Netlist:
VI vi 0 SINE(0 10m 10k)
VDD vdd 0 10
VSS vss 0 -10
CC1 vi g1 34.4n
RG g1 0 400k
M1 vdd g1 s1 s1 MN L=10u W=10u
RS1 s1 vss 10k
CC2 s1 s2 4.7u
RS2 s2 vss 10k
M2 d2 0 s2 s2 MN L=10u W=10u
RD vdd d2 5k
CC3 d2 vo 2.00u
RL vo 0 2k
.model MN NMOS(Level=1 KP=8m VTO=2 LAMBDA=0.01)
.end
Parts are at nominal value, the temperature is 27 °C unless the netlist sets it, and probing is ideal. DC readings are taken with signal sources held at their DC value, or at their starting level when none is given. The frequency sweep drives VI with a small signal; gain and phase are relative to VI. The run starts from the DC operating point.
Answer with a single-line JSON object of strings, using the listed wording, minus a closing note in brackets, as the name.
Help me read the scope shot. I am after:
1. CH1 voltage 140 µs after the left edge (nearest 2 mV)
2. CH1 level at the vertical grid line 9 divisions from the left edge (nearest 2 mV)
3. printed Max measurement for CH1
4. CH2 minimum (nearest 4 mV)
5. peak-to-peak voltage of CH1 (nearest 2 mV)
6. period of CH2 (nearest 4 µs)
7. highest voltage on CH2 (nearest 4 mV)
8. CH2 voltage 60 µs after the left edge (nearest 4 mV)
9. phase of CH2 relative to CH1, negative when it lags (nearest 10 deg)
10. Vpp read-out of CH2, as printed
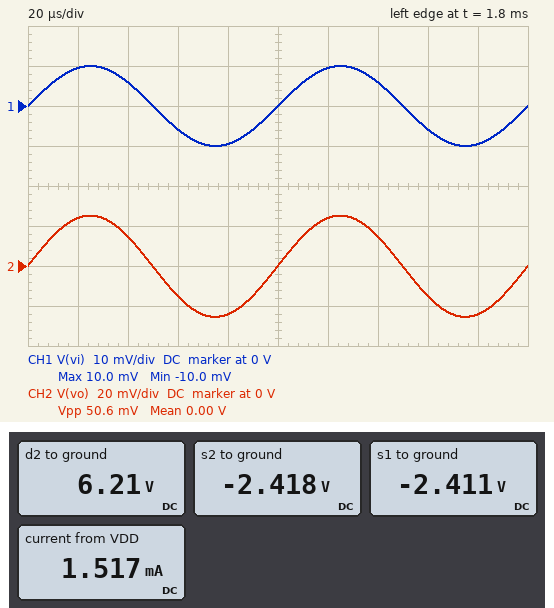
{"CH1 voltage 140 µs after the left edge": "6 mV", "CH1 level at the vertical grid line 9 divisions from the left edge": "-10 mV", "printed Max measurement for CH1": "10.0 mV", "CH2 minimum": "-24 mV", "peak-to-peak voltage of CH1": "20 mV", "period of CH2": "100 µs", "highest voltage on CH2": "24 mV", "CH2 voltage 60 µs after the left edge": "-16 mV", "phase of CH2 relative to CH1, negative when it lags": "0 deg", "Vpp read-out of CH2, as printed": "50.6 mV"}
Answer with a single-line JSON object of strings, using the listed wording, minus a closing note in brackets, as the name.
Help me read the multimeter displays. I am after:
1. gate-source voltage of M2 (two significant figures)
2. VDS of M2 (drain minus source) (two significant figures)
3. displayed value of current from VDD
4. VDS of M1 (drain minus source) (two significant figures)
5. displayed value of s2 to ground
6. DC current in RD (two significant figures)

{"gate-source voltage of M2": "2.4 V", "VDS of M2 (drain minus source)": "8.6 V", "displayed value of current from VDD": "1.517 mA", "VDS of M1 (drain minus source)": "12 V", "displayed value of s2 to ground": "-2.418 V", "DC current in RD": "760 µA"}
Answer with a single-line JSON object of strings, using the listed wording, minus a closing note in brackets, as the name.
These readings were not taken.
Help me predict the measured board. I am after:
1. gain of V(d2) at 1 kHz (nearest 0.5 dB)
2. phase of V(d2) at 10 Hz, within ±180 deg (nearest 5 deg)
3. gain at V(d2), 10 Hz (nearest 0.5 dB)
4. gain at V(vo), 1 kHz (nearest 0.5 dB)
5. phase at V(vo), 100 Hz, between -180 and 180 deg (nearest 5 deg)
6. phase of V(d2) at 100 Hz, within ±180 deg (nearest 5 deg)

{"gain of V(d2) at 1 kHz": "8.0 dB", "phase of V(d2) at 10 Hz, within ±180 deg": "105 deg", "gain at V(d2), 10 Hz": "-3.0 dB", "gain at V(vo), 1 kHz": "8.0 dB", "phase at V(vo), 100 Hz, between -180 and 180 deg": "45 deg", "phase of V(d2) at 100 Hz, within ±180 deg": "25 deg"}
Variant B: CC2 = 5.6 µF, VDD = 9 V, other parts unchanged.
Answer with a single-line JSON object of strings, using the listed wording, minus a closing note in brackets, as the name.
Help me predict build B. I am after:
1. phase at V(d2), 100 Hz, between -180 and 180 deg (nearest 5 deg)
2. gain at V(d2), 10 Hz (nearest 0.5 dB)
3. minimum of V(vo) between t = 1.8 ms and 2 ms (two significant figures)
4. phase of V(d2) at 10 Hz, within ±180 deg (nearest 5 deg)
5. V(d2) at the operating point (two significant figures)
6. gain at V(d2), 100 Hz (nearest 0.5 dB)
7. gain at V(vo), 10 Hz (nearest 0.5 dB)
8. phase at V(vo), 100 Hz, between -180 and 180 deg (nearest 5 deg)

{"phase at V(d2), 100 Hz, between -180 and 180 deg": "20 deg", "gain at V(d2), 10 Hz": "-1.5 dB", "minimum of V(vo) between t = 1.8 ms and 2 ms": "-25 mV", "phase of V(d2) at 10 Hz, within ±180 deg": "100 deg", "V(d2) at the operating point": "5.2 V", "gain at V(d2), 100 Hz": "7.5 dB", "gain at V(vo), 10 Hz": "-14.0 dB", "phase at V(vo), 100 Hz, between -180 and 180 deg": "40 deg"}
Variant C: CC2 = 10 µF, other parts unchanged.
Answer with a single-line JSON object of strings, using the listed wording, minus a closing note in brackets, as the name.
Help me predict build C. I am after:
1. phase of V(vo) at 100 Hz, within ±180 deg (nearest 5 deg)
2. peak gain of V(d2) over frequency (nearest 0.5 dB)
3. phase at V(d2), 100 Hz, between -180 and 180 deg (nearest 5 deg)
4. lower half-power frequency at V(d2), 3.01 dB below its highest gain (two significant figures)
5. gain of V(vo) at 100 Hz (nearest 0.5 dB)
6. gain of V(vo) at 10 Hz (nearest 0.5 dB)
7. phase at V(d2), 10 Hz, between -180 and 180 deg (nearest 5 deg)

{"phase of V(vo) at 100 Hz, within ±180 deg": "30 deg", "peak gain of V(d2) over frequency": "8.5 dB", "phase at V(d2), 100 Hz, between -180 and 180 deg": "10 deg", "lower half-power frequency at V(d2), 3.01 dB below its highest gain": "13 Hz", "gain of V(vo) at 100 Hz": "7.5 dB", "gain of V(vo) at 10 Hz": "-9.0 dB", "phase at V(d2), 10 Hz, between -180 and 180 deg": "95 deg"}
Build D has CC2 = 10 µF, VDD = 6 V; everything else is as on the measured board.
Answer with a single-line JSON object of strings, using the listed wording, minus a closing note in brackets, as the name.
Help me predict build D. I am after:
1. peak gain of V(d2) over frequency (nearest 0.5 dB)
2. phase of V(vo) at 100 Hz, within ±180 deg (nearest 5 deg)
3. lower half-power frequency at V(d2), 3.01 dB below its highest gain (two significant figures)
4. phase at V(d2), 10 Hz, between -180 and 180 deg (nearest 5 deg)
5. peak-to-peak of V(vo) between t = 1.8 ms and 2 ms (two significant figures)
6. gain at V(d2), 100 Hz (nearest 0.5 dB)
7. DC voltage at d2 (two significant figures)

{"peak gain of V(d2) over frequency": "8.5 dB", "phase of V(vo) at 100 Hz, within ±180 deg": "30 deg", "lower half-power frequency at V(d2), 3.01 dB below its highest gain": "13 Hz", "phase at V(d2), 10 Hz, between -180 and 180 deg": "95 deg", "peak-to-peak of V(vo) between t = 1.8 ms and 2 ms": "50 mV", "gain at V(d2), 100 Hz": "8.0 dB", "DC voltage at d2": "2.2 V"}
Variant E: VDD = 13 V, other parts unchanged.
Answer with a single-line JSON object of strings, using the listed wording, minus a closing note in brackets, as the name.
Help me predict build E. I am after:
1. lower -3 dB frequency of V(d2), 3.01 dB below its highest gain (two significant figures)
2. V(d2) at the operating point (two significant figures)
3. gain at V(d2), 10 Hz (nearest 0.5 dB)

{"lower -3 dB frequency of V(d2), 3.01 dB below its highest gain": "43 Hz", "V(d2) at the operating point": "9.2 V", "gain at V(d2), 10 Hz": "-3.0 dB"}
